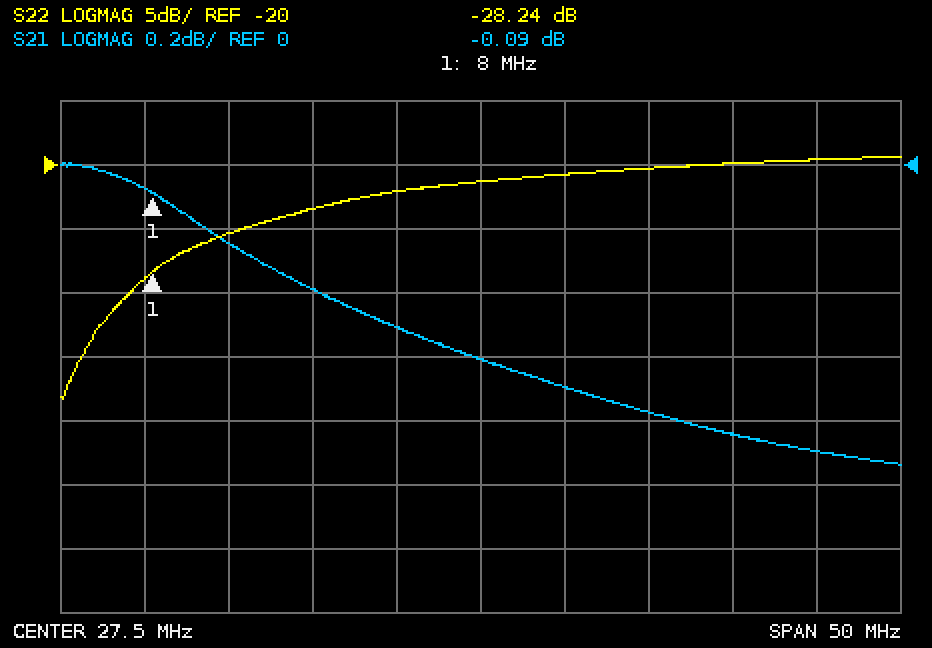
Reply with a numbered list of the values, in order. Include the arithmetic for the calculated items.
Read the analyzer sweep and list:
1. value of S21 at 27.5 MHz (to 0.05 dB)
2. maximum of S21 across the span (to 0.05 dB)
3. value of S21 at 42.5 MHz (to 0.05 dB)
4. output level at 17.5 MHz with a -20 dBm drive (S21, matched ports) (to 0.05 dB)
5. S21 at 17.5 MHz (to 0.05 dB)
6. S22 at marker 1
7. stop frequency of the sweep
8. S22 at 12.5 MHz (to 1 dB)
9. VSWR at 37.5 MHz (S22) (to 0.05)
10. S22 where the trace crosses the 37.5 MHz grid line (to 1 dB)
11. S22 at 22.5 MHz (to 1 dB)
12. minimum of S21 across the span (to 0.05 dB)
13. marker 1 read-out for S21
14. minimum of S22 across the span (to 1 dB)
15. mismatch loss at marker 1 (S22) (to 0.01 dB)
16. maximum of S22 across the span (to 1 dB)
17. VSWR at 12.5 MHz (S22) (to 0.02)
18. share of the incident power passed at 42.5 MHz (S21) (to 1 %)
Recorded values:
1. -0.60 dB
2. 0.00 dB
3. -0.85 dB
4. -20 dBm + (-0.40 dB) = -20.40 dBm
5. -0.40 dB
6. -28.24 dB
7. 52.5 MHz
8. -25 dB
9. |Γ| = 10^(-20/20) = 0.1000; VSWR = (1 + 0.1000)/(1 − 0.1000) ≈ 1.22, so 1.20 to the nearest 0.05
10. -20 dB
11. -22 dB
12. -0.95 dB
13. -0.09 dB
14. -38 dB
15. −10 log10(1 − 10^(-28.24/10)) ≈ 0.01 dB
16. -19 dB
17. |Γ| = 10^(-25/20) = 0.0562; VSWR = (1 + 0.0562)/(1 − 0.0562) ≈ 1.12
18. 10^(-0.85/10) ≈ 82 %
